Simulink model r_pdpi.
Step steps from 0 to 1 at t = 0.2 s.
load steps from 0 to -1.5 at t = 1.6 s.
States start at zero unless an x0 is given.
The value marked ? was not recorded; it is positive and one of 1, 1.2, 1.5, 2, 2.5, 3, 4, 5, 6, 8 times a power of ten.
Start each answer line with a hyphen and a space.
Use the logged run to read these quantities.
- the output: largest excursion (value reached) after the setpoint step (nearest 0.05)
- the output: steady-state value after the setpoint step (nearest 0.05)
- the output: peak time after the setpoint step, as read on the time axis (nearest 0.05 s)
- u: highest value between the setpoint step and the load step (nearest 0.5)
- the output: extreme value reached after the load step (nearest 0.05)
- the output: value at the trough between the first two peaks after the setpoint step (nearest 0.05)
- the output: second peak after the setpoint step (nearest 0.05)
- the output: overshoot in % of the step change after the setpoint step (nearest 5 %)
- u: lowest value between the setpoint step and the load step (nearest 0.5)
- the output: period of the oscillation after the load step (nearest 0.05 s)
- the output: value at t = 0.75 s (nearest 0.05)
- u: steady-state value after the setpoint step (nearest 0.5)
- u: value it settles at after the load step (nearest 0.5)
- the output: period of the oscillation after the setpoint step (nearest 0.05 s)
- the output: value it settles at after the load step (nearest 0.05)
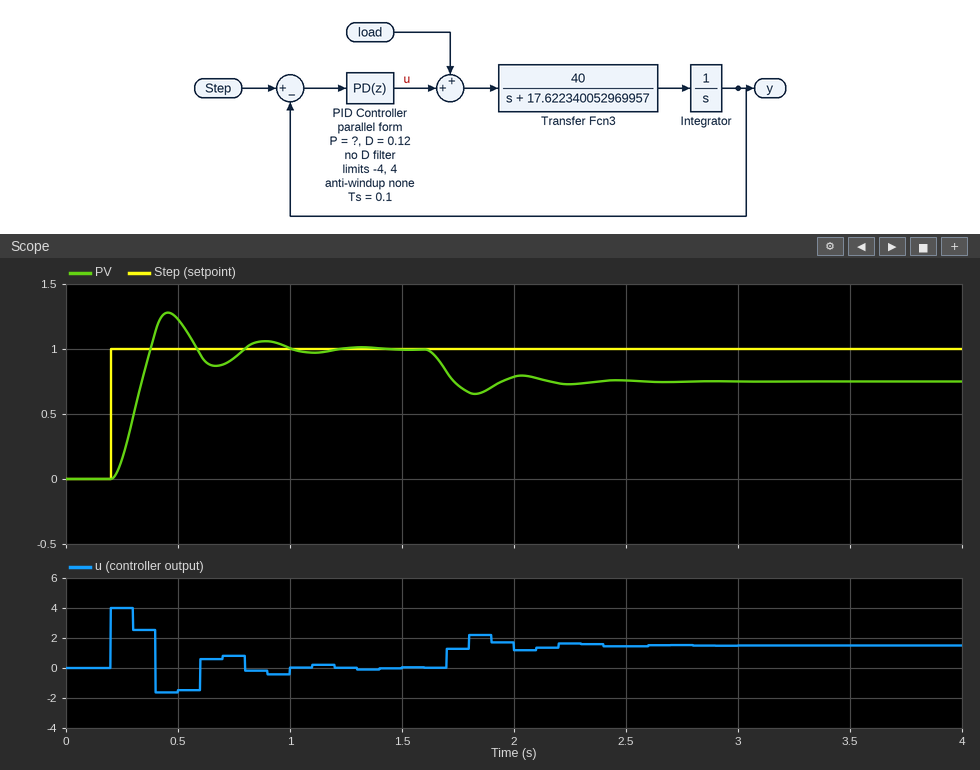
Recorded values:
- 1.30
- 1.00
- 0.45 s
- 4.0
- 0.65
- 0.85
- 1.05
- 30 %
- -1.5
- 0.40 s
- 0.95
- 0.0
- 1.5
- 0.45 s
- 0.75
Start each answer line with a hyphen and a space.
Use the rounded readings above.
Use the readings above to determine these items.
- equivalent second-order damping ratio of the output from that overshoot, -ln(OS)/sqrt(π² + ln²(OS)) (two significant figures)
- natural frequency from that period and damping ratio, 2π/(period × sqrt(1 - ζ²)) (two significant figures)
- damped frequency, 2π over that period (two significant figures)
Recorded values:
- 0.36
- 15 rad/s
- 14 rad/s
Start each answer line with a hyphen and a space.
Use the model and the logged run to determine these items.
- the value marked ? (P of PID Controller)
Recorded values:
- 6
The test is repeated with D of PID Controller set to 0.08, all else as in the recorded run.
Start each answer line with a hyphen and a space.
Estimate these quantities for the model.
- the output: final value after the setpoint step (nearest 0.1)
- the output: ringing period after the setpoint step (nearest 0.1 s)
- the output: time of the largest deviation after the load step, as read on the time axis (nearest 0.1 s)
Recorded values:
- 1.0
- 0.5 s
- 1.8 s
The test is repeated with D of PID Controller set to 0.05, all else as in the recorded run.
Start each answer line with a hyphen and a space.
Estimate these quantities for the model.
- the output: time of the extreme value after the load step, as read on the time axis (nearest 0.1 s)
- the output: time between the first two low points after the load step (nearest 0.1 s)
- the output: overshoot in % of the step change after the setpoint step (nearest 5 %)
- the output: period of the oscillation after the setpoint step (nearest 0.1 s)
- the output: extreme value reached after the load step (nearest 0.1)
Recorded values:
- 1.8 s
- 0.5 s
- 35 %
- 0.5 s
- 0.6
